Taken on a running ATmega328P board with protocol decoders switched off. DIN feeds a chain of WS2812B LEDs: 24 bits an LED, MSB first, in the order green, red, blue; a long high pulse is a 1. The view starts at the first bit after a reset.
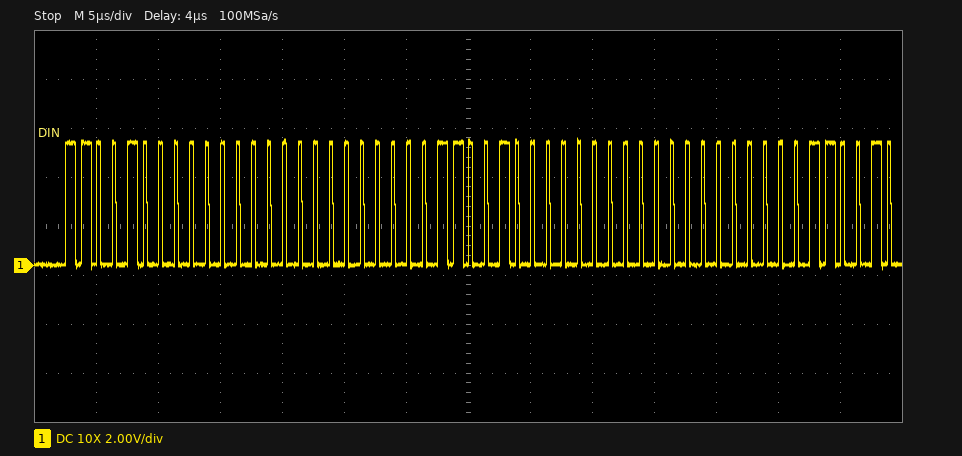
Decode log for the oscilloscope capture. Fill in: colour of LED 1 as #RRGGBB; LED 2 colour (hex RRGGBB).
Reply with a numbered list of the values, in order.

1. #00C800
2. #00C800
